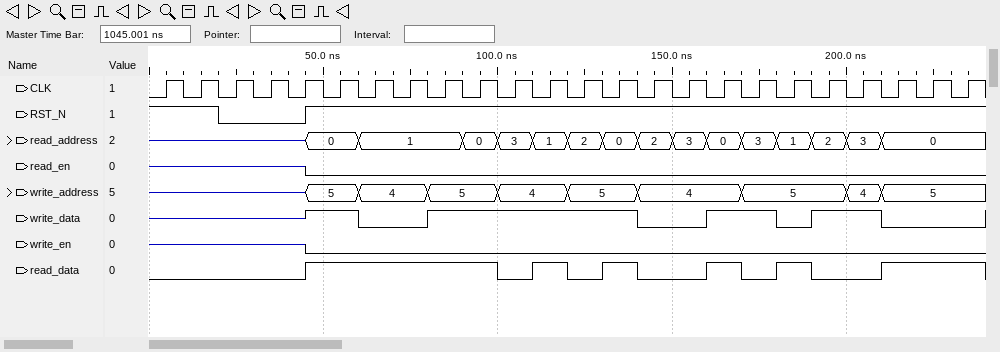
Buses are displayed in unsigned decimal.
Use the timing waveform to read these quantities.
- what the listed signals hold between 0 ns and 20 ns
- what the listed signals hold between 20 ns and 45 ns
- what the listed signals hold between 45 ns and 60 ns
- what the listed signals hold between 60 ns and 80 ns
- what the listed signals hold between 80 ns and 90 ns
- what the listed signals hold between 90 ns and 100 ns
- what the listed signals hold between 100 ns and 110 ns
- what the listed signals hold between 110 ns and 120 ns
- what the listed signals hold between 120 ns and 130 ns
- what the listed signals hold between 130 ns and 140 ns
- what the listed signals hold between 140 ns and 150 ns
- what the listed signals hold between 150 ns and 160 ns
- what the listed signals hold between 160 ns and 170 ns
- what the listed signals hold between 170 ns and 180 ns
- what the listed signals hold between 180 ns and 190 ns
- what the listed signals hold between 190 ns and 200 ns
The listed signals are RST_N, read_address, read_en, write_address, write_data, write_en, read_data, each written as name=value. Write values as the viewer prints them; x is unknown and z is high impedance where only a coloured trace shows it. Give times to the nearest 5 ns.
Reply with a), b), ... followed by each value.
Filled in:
a) RST_N=1, read_address=z, read_en=z, write_address=z, write_data=z, write_en=z, read_data=0
b) RST_N=0, read_address=z, read_en=z, write_address=z, write_data=z, write_en=z, read_data=0
c) RST_N=1, read_address=0, read_en=0, write_address=5, write_data=1, write_en=0, read_data=1
d) RST_N=1, read_address=1, read_en=0, write_address=4, write_data=0, write_en=0, read_data=1
e) RST_N=1, read_address=1, read_en=0, write_address=5, write_data=1, write_en=0, read_data=1
f) RST_N=1, read_address=0, read_en=0, write_address=5, write_data=1, write_en=0, read_data=1
g) RST_N=1, read_address=3, read_en=0, write_address=4, write_data=1, write_en=0, read_data=0
h) RST_N=1, read_address=1, read_en=0, write_address=4, write_data=1, write_en=0, read_data=1
i) RST_N=1, read_address=2, read_en=0, write_address=5, write_data=1, write_en=0, read_data=0
j) RST_N=1, read_address=0, read_en=0, write_address=5, write_data=1, write_en=0, read_data=1
k) RST_N=1, read_address=2, read_en=0, write_address=4, write_data=0, write_en=0, read_data=0
l) RST_N=1, read_address=3, read_en=0, write_address=4, write_data=0, write_en=0, read_data=0
m) RST_N=1, read_address=0, read_en=0, write_address=4, write_data=1, write_en=0, read_data=1
n) RST_N=1, read_address=3, read_en=0, write_address=5, write_data=1, write_en=0, read_data=0
o) RST_N=1, read_address=1, read_en=0, write_address=5, write_data=0, write_en=0, read_data=1
p) RST_N=1, read_address=2, read_en=0, write_address=5, write_data=1, write_en=0, read_data=0
